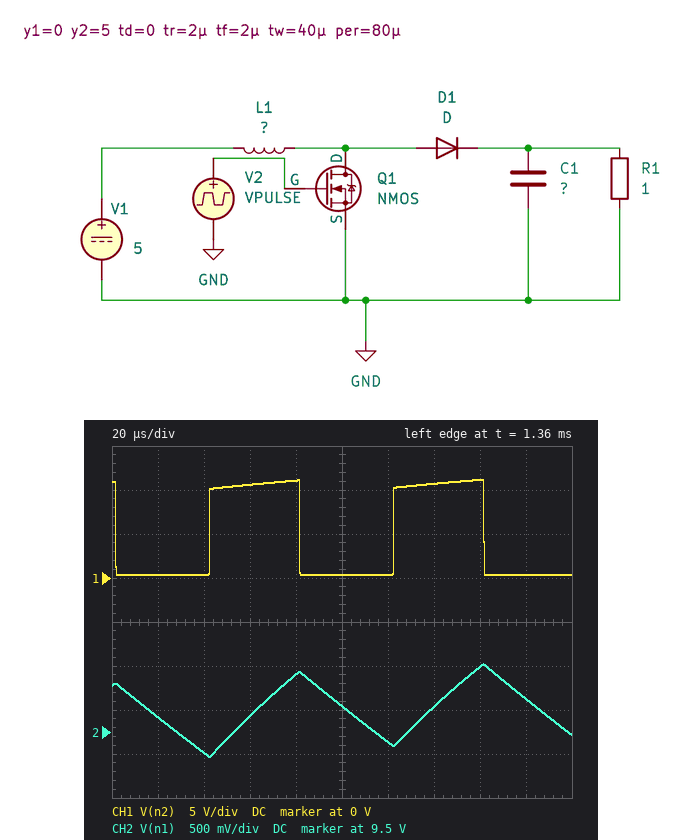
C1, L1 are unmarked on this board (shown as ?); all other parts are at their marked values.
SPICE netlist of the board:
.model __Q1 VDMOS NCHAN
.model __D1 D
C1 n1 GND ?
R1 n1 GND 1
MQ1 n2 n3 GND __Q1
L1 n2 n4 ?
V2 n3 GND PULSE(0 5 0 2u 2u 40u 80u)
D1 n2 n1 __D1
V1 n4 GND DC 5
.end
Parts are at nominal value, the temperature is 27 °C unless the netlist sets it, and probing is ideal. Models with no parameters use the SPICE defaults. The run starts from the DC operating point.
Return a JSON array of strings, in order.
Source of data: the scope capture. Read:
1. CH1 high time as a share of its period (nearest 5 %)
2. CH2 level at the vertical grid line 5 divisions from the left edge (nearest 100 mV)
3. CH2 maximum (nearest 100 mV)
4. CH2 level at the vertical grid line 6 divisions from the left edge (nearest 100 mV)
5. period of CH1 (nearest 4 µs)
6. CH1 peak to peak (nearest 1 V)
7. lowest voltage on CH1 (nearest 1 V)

["50 %", "9.8 V", "10.3 V", "9.4 V", "80 µs", "11 V", "0 V"]
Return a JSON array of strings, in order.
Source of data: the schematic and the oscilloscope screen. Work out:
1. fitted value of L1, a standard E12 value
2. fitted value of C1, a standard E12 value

["100 µH", "470 µF"]
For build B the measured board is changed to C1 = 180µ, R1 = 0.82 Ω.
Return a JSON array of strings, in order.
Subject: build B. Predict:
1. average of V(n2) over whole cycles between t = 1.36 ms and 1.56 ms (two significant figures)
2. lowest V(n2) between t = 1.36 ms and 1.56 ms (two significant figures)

["5.0 V", "330 mV"]
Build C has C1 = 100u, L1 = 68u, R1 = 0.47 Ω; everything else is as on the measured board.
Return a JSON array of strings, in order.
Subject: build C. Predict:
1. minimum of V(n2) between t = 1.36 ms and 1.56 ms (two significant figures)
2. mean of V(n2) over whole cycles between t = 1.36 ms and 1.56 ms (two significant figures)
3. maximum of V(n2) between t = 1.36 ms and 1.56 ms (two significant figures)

["530 mV", "4.8 V", "12 V"]
